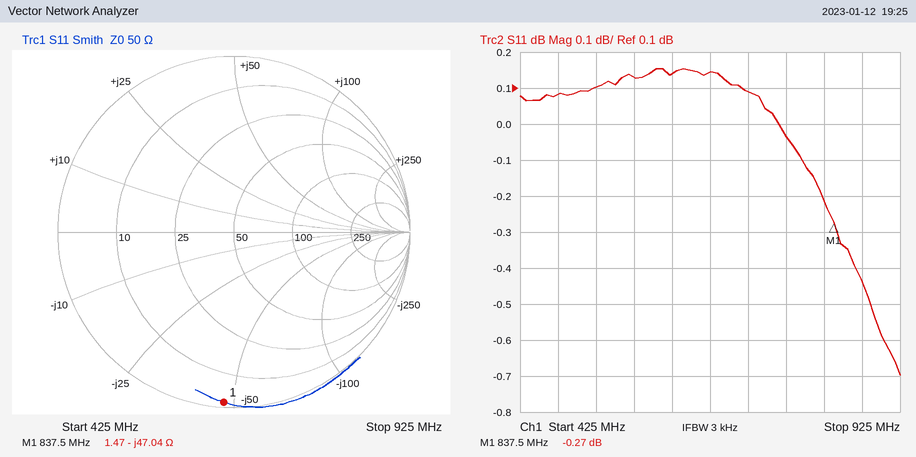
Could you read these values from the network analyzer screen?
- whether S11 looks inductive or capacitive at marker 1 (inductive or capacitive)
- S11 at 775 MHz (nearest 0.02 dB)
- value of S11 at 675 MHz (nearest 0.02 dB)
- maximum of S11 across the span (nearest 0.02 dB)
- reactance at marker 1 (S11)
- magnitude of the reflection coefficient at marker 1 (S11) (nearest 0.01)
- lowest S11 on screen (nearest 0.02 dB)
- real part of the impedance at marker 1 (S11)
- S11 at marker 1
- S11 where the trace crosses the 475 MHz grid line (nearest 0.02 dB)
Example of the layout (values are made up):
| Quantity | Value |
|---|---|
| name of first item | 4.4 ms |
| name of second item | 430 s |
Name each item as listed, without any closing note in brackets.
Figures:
| Quantity | Value |
|---|---|
| whether S11 looks inductive or capacitive at marker 1 | capacitive |
| S11 at 775 MHz | -0.04 dB |
| value of S11 at 675 MHz | 0.14 dB |
| maximum of S11 across the span | 0.16 dB |
| reactance at marker 1 | -47.04 Ω |
| magnitude of the reflection coefficient at marker 1 (S11) | 0.97 |
| lowest S11 on screen | -0.70 dB |
| real part of the impedance at marker 1 | 1.47 Ω |
| S11 at marker 1 | -0.27 dB |
| S11 where the trace crosses the 475 MHz grid line | 0.08 dB |
